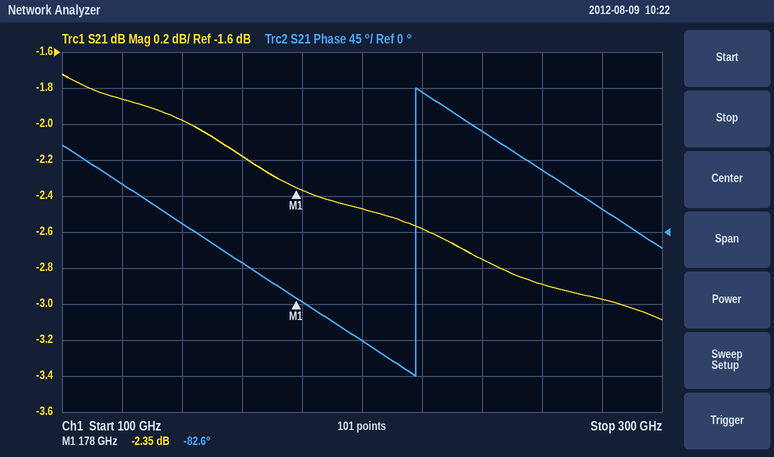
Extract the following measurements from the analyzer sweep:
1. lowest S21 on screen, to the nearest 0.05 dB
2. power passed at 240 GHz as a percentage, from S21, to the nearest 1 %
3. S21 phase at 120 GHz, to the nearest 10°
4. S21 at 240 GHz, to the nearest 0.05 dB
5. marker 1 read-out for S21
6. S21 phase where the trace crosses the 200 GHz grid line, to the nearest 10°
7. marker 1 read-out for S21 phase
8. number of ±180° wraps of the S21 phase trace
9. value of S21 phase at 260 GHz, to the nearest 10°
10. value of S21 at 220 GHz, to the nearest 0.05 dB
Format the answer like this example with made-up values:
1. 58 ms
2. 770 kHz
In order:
1. -3.10 dB
2. 53 %
3. 60°
4. -2.75 dB
5. -2.35 dB
6. -140°
7. -82.6°
8. 1
9. 80°
10. -2.60 dB
